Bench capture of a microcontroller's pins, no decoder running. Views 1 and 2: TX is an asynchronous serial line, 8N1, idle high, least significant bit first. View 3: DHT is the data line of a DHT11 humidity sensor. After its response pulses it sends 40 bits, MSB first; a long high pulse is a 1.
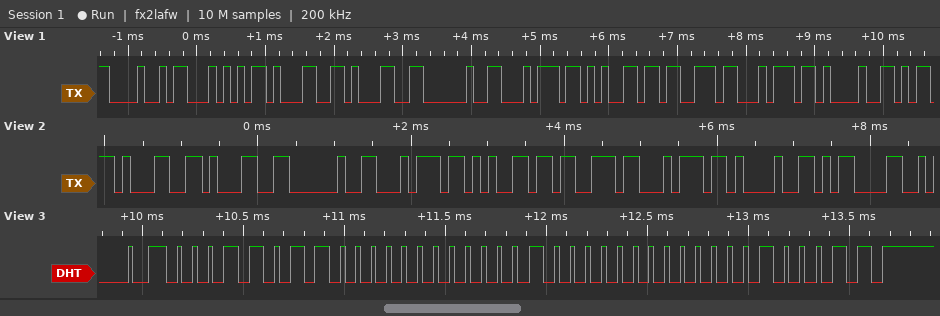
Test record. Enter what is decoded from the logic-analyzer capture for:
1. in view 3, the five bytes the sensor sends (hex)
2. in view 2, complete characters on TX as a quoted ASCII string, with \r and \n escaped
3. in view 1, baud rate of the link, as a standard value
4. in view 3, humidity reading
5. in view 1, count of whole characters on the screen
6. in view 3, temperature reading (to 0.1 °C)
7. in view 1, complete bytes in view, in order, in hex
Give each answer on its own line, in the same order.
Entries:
1B 00 08 00 23
"11 test!\r"
9600 baud
27 %
10
8.0 °C
48 54 31 31 20 74 65 73 74 21
